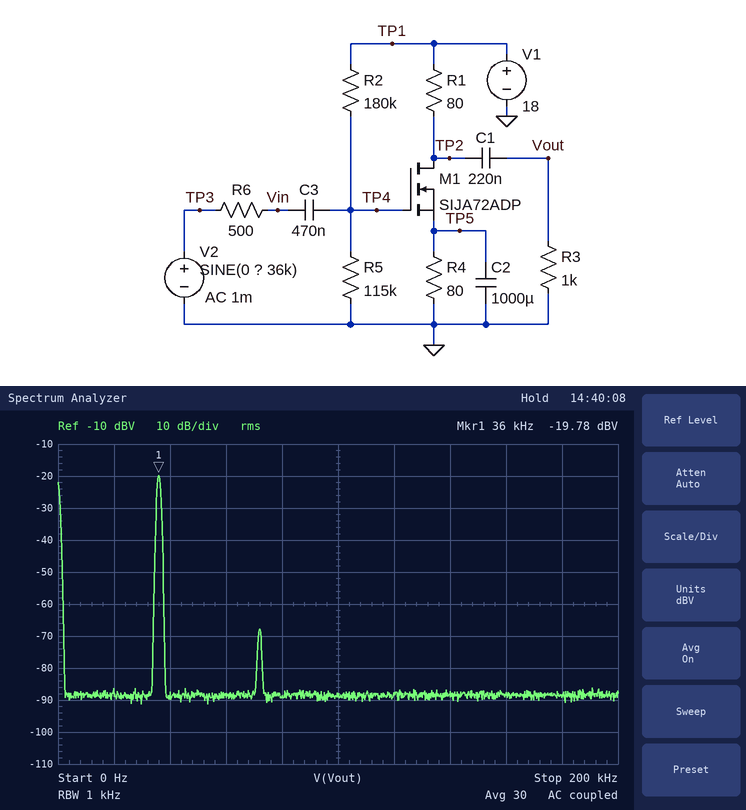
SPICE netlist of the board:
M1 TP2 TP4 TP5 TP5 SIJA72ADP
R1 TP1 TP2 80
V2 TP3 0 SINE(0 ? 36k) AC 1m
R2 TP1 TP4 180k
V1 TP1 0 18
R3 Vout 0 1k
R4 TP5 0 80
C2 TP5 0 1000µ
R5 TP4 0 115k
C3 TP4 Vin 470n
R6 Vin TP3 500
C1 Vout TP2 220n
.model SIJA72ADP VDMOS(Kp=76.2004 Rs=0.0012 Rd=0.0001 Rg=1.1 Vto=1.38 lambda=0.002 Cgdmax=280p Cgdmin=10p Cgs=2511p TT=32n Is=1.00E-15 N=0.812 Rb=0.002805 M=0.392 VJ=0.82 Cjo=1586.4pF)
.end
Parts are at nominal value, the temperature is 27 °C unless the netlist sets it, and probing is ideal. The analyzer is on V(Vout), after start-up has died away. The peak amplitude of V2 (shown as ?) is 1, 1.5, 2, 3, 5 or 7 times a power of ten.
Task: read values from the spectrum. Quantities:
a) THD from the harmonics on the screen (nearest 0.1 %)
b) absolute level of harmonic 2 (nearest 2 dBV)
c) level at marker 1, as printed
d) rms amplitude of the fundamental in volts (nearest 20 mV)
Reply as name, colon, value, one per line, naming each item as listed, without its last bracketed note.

THD from the harmonics on the screen: 0.4 %
absolute level of harmonic 2: -68 dBV
level at marker 1, as printed: -19.78 dBV
rms amplitude of the fundamental in volts: 100 mV
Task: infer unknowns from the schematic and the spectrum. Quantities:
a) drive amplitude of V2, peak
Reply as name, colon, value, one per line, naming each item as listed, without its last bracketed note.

drive amplitude of V2, peak: 2 mV
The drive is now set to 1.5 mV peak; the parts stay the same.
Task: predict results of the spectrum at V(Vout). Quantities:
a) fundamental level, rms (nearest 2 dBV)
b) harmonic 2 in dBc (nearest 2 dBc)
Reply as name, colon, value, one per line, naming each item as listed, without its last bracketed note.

fundamental level, rms: -22 dBV
harmonic 2 in dBc: -50 dBc
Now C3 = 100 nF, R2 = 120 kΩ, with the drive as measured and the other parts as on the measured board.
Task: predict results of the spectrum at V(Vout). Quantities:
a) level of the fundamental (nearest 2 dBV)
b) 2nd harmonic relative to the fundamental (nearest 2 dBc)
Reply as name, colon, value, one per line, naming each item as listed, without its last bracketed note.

level of the fundamental: -20 dBV
2nd harmonic relative to the fundamental: -42 dBc
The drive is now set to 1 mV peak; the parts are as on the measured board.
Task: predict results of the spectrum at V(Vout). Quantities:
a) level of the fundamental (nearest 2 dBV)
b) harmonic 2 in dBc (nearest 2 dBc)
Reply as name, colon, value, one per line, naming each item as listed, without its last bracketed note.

level of the fundamental: -26 dBV
harmonic 2 in dBc: -54 dBc
